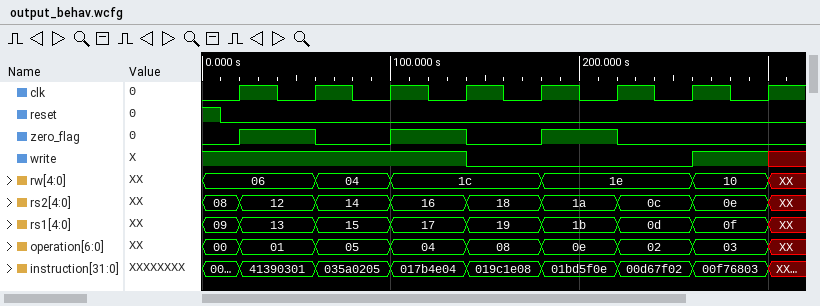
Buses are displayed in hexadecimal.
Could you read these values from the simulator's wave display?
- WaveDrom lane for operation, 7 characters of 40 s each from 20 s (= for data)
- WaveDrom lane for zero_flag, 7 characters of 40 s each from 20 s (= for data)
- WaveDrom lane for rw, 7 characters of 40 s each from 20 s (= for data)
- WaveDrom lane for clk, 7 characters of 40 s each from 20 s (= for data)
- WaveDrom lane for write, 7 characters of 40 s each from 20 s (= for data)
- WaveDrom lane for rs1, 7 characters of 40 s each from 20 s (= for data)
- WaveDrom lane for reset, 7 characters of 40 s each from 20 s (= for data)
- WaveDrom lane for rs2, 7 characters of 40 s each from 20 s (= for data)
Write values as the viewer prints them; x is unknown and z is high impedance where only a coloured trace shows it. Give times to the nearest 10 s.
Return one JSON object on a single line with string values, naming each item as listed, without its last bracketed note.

{"WaveDrom lane for operation, 7 characters of 40 s each from 20 s": "{name: 'operation', wave: '=======', data: '01 05 04 08 0e 02 03'}", "WaveDrom lane for zero_flag, 7 characters of 40 s each from 20 s": "{name: 'zero_flag', wave: '101010.'}", "WaveDrom lane for rw, 7 characters of 40 s each from 20 s": "{name: 'rw', wave: '===.=.=', data: '06 04 1c 1e 10'}", "WaveDrom lane for clk, 7 characters of 40 s each from 20 s": "{name: 'clk', wave: 'p......'}", "WaveDrom lane for write, 7 characters of 40 s each from 20 s": "{name: 'write', wave: '1..0..1'}", "WaveDrom lane for rs1, 7 characters of 40 s each from 20 s": "{name: 'rs1', wave: '=======', data: '13 15 17 19 1b 0d 0f'}", "WaveDrom lane for reset, 7 characters of 40 s each from 20 s": "{name: 'reset', wave: '0......'}", "WaveDrom lane for rs2, 7 characters of 40 s each from 20 s": "{name: 'rs2', wave: '=======', data: '12 14 16 18 1a 0c 0e'}"}
